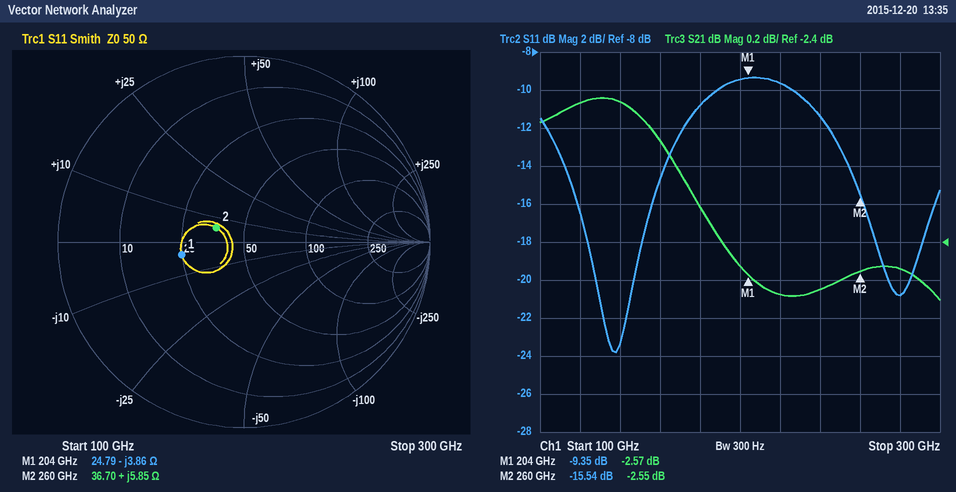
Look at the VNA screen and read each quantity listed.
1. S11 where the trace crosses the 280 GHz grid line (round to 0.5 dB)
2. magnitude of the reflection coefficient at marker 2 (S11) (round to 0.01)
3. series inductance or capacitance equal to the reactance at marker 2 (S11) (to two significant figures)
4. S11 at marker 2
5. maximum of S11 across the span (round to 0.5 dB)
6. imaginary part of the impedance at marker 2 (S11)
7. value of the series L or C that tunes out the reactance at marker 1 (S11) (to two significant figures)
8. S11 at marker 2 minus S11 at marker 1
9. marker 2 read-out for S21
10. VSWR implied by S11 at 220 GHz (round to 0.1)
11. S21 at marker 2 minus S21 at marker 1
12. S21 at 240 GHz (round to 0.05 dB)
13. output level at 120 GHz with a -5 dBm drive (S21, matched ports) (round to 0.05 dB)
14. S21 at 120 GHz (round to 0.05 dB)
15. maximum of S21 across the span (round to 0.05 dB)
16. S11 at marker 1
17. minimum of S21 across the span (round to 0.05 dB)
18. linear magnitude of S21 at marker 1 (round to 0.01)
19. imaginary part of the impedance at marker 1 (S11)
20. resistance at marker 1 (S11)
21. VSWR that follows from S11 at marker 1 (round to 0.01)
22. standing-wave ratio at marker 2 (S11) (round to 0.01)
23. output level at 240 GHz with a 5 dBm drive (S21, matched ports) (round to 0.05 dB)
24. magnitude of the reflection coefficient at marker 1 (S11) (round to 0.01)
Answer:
-21.0 dB
0.17
3.6 pH
-15.54 dB
-9.5 dB
+5.85 Ω
3.0 pH
-6.19 dB
-2.55 dB
2.0
0.02 dB
-2.65 dB
-6.65 dBm
-1.65 dB
-1.65 dB
-9.35 dB
-2.70 dB
0.74
-3.86 Ω
24.79 Ω
2.03
1.40
2.35 dBm
0.34
